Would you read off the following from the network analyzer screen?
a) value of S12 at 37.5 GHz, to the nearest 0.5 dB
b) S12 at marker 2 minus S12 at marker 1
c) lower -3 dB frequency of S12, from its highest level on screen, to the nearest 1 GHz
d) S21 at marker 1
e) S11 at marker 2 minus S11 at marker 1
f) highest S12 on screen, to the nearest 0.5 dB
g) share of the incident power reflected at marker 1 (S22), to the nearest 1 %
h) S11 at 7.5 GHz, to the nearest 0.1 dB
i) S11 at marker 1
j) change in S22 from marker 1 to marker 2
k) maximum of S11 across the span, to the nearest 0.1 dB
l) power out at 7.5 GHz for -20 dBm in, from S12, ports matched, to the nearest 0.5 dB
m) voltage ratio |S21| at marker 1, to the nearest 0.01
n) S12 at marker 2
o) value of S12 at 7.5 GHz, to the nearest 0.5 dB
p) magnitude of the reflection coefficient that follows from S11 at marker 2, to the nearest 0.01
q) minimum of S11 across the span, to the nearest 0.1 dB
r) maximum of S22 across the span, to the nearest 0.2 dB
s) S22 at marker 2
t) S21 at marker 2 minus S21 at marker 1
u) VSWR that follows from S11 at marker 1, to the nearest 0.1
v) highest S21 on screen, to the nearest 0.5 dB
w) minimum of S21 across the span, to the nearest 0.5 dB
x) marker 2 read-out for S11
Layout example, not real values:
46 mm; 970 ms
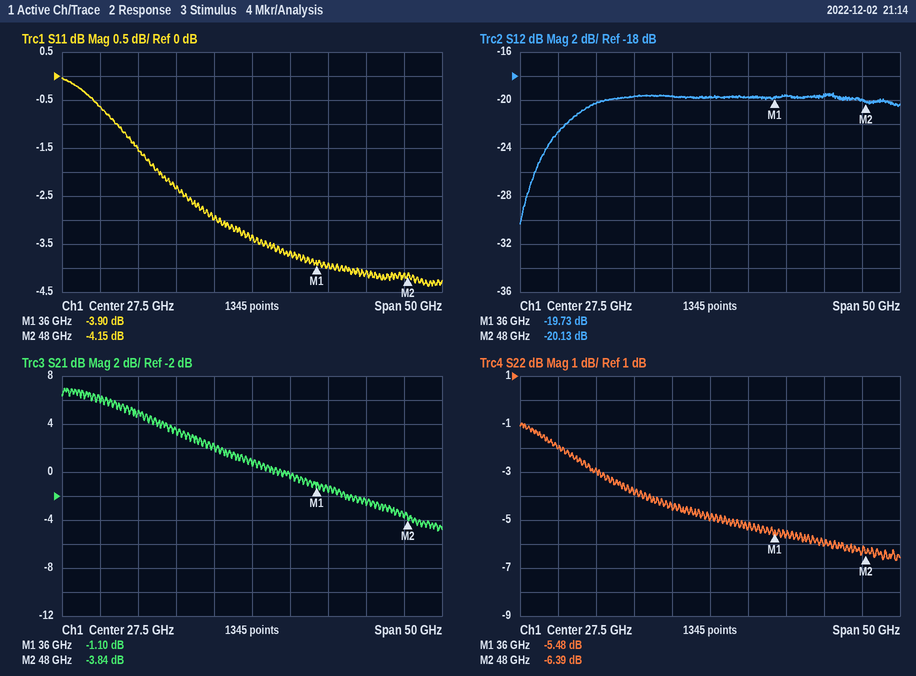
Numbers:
-19.5 dB; -0.40 dB; 8 GHz; -1.10 dB; -0.25 dB; -19.5 dB; 28 %; -0.6 dB; -3.90 dB; -0.91 dB; 0.0 dB; -42.5 dBm; 0.88; -20.13 dB; -22.5 dB; 0.62; -4.4 dB; -1.0 dB; -6.39 dB; -2.74 dB; 4.5; 7.0 dB; -5.0 dB; -4.15 dB
